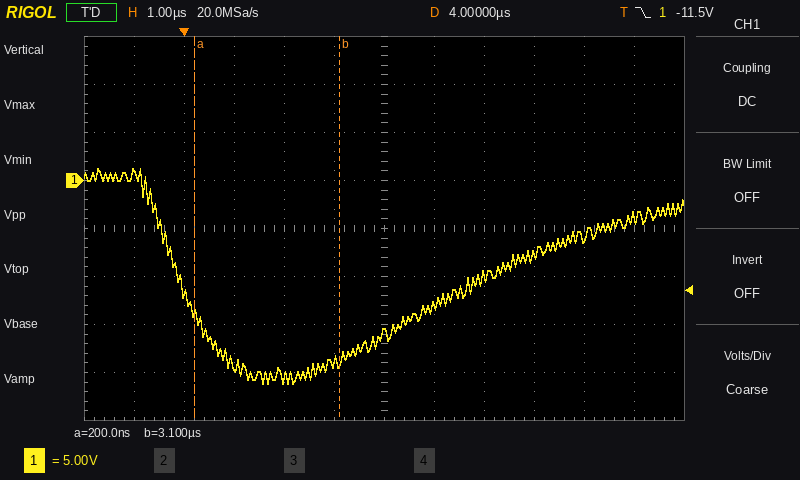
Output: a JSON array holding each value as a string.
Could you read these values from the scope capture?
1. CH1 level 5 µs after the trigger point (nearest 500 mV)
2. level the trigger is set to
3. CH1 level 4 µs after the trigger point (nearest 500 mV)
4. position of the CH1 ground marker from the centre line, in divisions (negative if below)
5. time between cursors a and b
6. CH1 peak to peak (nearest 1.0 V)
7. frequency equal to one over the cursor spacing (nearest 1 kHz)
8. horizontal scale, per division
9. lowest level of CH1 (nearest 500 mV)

["-13.0 V", "-11.5 V", "-16.0 V", "+1.0 div", "2.9 µs", "22.0 V", "345 kHz", "1 µs", "-21.0 V"]
